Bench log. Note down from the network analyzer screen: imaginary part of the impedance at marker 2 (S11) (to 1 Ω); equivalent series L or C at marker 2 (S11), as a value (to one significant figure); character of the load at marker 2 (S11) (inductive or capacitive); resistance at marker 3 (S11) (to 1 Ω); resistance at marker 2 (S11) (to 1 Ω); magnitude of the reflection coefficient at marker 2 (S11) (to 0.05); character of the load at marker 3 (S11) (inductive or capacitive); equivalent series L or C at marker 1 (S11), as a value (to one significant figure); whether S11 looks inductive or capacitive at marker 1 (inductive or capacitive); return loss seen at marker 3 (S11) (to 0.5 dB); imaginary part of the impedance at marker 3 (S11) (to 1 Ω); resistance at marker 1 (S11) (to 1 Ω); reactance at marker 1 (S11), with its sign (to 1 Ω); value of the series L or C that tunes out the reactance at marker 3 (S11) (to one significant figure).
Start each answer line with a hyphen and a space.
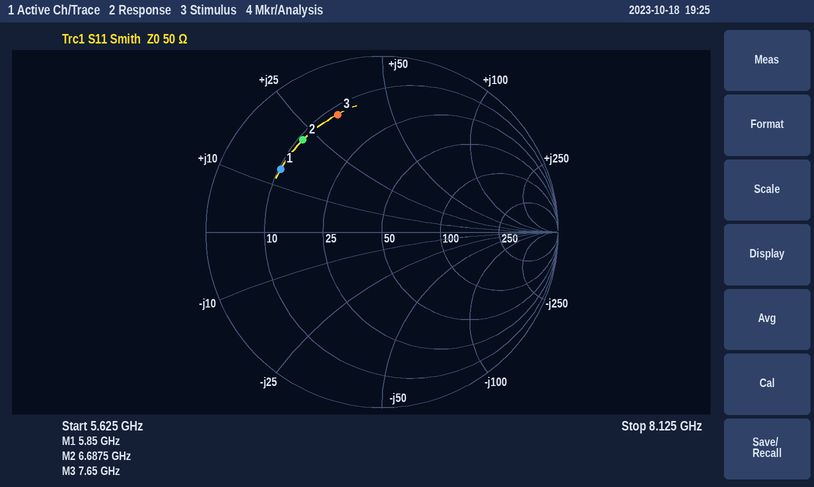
- +22 Ω
- 500 pH
- inductive
- 12 Ω
- 11 Ω
- 0.70
- inductive
- 400 pH
- inductive
- 3.0 dB
- +33 Ω
- 10 Ω
- +14 Ω
- 600 fF
